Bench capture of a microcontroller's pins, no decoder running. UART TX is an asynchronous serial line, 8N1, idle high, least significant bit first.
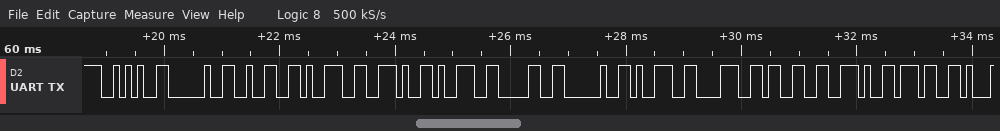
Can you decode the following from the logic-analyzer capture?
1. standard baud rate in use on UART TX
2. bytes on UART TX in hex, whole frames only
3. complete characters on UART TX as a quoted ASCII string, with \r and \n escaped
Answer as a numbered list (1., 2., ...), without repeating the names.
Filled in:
1. 9600 baud
2. 2A 20 32 39 2E 39 30 20 39 38 33 2E 37
3. "* 29.90 983.7"
